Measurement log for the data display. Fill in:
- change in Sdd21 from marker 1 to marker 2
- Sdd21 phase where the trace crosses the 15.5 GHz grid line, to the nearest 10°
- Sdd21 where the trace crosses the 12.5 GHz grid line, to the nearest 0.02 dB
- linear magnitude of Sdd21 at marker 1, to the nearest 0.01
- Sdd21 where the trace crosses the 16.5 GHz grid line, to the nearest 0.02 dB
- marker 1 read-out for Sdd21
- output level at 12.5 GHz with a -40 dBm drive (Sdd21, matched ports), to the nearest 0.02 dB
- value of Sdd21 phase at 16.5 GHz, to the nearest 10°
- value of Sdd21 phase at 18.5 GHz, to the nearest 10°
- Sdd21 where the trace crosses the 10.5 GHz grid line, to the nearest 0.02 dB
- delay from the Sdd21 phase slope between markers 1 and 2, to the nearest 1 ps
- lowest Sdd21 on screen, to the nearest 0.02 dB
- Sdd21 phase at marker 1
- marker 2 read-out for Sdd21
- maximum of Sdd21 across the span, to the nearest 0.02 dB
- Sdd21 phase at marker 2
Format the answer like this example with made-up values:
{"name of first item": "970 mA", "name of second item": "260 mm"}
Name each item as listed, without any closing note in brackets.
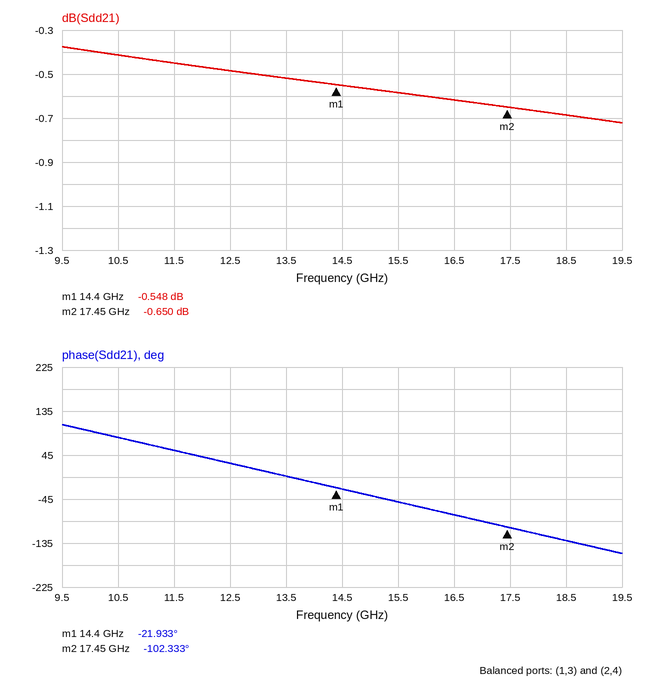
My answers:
{"change in Sdd21 from marker 1 to marker 2": "-0.102 dB", "Sdd21 phase where the trace crosses the 15.5 GHz grid line, to the nearest 10°": "-50°", "Sdd21 where the trace crosses the 12.5 GHz grid line, to the nearest 0.02 dB": "-0.48 dB", "linear magnitude of Sdd21 at marker 1, to the nearest 0.01": "0.94", "Sdd21 where the trace crosses the 16.5 GHz grid line, to the nearest 0.02 dB": "-0.62 dB", "marker 1 read-out for Sdd21": "-0.548 dB", "output level at 12.5 GHz with a -40 dBm drive (Sdd21, matched ports), to the nearest 0.02 dB": "-40.48 dBm", "value of Sdd21 phase at 16.5 GHz, to the nearest 10°": "-80°", "value of Sdd21 phase at 18.5 GHz, to the nearest 10°": "-130°", "Sdd21 where the trace crosses the 10.5 GHz grid line, to the nearest 0.02 dB": "-0.42 dB", "delay from the Sdd21 phase slope between markers 1 and 2, to the nearest 1 ps": "73 ps", "lowest Sdd21 on screen, to the nearest 0.02 dB": "-0.72 dB", "Sdd21 phase at marker 1": "-21.933°", "marker 2 read-out for Sdd21": "-0.650 dB", "maximum of Sdd21 across the span, to the nearest 0.02 dB": "-0.38 dB", "Sdd21 phase at marker 2": "-102.333°"}
